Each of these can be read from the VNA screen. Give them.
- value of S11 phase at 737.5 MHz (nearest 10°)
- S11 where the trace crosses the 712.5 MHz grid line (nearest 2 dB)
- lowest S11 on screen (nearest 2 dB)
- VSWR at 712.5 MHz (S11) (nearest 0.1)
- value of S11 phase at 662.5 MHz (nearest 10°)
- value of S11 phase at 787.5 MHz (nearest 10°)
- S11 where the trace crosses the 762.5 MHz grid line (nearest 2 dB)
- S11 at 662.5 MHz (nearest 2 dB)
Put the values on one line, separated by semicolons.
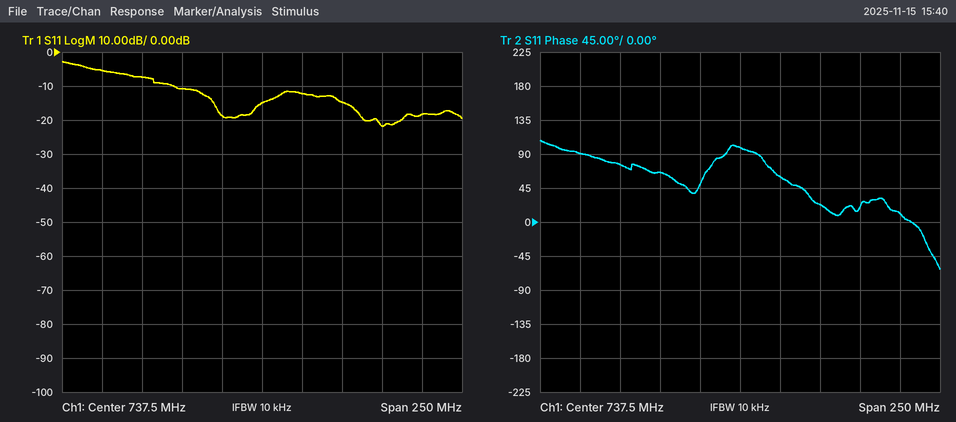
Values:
100°; -18 dB; -22 dB; 1.3; 80°; 20°; -12 dB; -8 dB
